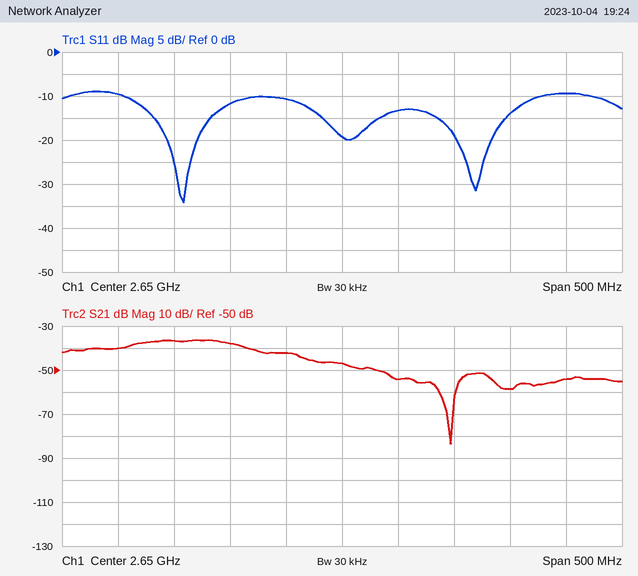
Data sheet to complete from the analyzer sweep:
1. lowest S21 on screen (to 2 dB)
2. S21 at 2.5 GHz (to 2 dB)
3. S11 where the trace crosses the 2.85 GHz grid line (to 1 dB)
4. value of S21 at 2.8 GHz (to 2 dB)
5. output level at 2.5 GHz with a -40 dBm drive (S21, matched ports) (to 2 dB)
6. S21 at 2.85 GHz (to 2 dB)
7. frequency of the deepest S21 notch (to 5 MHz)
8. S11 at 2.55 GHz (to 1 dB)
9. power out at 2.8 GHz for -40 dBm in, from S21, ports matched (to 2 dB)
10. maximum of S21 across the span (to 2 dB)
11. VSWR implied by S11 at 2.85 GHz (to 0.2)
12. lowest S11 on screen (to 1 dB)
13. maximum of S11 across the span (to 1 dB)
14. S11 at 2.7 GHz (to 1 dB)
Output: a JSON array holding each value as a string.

["-84 dB", "-36 dB", "-9 dB", "-58 dB", "-76 dBm", "-54 dB", "2.745 GHz", "-12 dB", "-98 dBm", "-36 dB", "2.0", "-34 dB", "-9 dB", "-13 dB"]
